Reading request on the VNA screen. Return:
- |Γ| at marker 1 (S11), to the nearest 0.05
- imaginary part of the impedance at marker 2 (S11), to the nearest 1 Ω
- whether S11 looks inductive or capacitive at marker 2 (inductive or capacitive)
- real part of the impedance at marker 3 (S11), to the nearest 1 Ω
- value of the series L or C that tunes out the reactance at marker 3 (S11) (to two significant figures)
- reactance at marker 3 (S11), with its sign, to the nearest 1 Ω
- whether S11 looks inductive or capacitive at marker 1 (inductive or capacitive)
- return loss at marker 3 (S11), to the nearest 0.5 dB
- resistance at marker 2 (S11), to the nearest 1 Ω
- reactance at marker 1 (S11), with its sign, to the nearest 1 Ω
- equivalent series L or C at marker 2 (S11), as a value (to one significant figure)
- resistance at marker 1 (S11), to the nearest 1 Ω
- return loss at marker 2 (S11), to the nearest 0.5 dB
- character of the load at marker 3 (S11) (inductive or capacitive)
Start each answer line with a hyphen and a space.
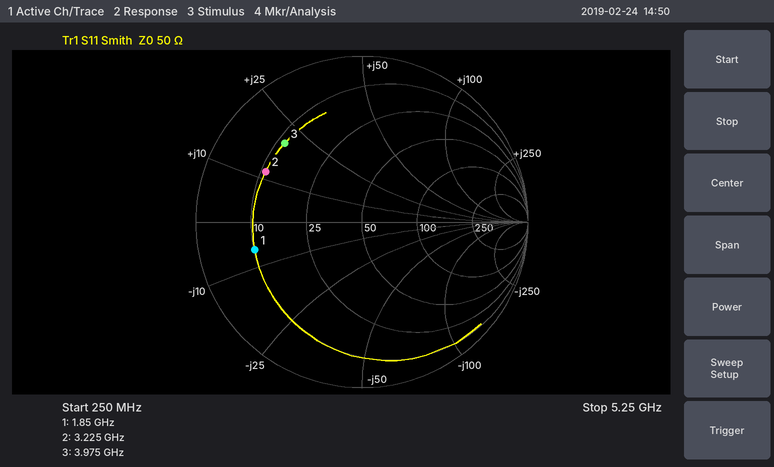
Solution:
- 0.65
- +12 Ω
- inductive
- 12 Ω
- 2.0 pF
- +20 Ω
- capacitive
- 3.5 dB
- 11 Ω
- -6 Ω
- 600 pH
- 10 Ω
- 3.5 dB
- inductive
